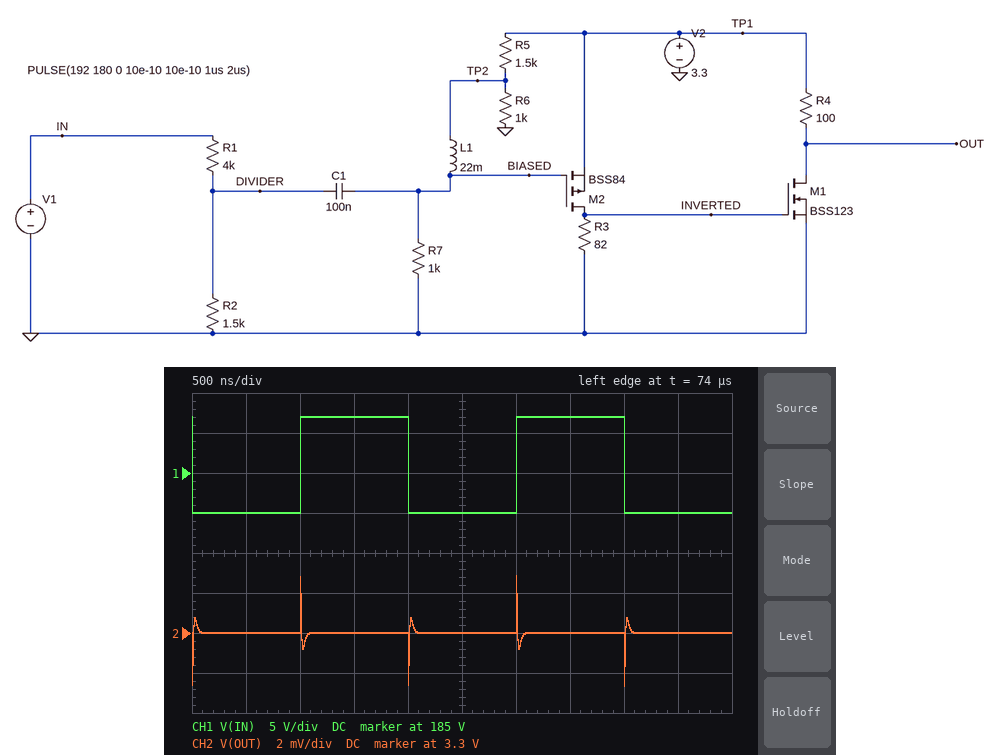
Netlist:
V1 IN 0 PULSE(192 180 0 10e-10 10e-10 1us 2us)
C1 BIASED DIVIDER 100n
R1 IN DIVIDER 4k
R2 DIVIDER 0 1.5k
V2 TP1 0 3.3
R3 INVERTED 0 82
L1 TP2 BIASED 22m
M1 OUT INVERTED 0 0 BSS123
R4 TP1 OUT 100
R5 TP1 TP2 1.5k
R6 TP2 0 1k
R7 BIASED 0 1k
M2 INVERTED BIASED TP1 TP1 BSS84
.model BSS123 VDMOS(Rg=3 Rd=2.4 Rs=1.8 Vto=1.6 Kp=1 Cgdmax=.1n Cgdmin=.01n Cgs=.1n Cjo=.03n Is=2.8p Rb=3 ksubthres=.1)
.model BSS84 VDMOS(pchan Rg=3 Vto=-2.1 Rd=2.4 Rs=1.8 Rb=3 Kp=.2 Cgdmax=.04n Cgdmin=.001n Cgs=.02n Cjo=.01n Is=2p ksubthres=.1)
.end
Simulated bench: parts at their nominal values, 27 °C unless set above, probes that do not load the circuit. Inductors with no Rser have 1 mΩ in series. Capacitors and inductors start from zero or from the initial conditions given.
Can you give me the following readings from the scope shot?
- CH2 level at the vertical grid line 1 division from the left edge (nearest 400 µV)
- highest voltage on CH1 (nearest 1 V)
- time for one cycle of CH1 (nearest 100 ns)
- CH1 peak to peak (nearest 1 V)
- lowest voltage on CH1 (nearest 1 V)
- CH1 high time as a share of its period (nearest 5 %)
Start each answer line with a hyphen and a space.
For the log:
- 3.3000 V
- 192 V
- 2.0 µs
- 12 V
- 180 V
- 50 %
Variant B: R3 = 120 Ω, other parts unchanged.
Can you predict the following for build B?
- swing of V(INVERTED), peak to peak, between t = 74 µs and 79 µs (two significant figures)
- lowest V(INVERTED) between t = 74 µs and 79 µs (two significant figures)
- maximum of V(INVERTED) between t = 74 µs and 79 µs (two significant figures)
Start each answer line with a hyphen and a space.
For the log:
- 30 mV
- -15 mV
- 15 mV
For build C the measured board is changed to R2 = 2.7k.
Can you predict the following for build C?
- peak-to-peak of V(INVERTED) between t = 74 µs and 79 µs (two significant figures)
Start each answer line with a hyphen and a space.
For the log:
- 23 mV
